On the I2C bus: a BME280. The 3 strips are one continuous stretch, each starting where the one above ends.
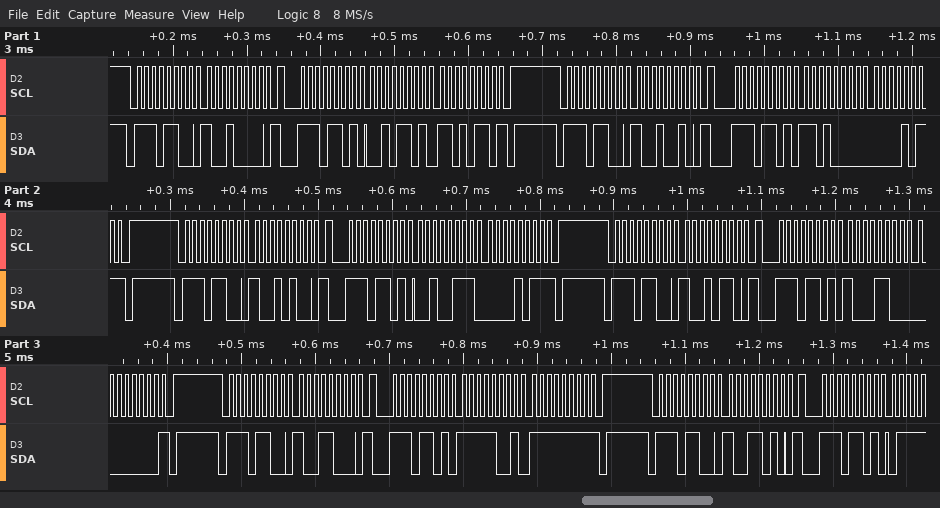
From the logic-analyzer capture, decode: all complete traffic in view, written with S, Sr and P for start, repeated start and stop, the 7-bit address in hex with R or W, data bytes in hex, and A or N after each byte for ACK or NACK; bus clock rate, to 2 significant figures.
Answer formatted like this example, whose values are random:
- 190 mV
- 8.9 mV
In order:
- S 76W A 90 A Sr 76R A 2D A D6 N P S 76W A 92 A Sr 76R A D0 A 0B N P S 76W A 94 A Sr 76R A 27 A 0B N P S 76W A 96 A Sr 76R A 8C A 00 N P S 76W A 98 A Sr 76R A F9 A FF N P S 76W A 9A A Sr 76R A
- 100 kHz
